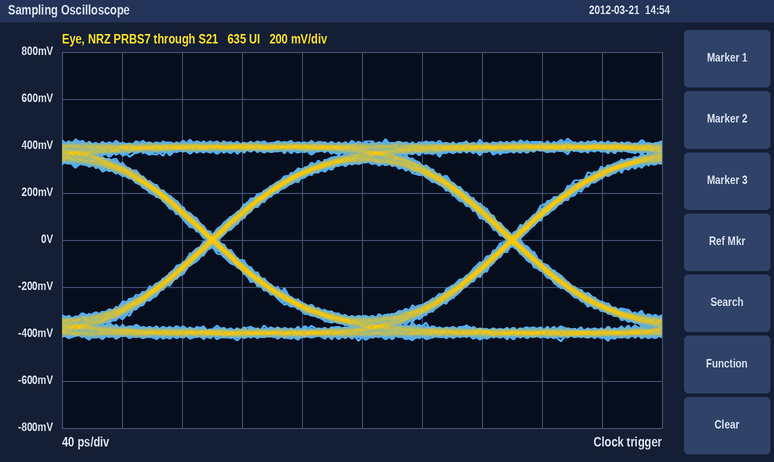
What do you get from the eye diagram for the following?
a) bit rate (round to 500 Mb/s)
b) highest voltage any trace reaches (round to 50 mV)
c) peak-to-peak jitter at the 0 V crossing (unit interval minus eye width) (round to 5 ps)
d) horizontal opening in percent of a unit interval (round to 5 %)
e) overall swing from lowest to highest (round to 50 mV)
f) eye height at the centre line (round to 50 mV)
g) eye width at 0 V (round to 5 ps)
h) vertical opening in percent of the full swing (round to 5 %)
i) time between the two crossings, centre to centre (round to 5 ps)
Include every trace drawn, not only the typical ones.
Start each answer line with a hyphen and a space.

- 5.0 Gb/s
- 450 mV
- 10 ps
- 95 %
- 850 mV
- 650 mV
- 190 ps
- 75 %
- 200 ps
